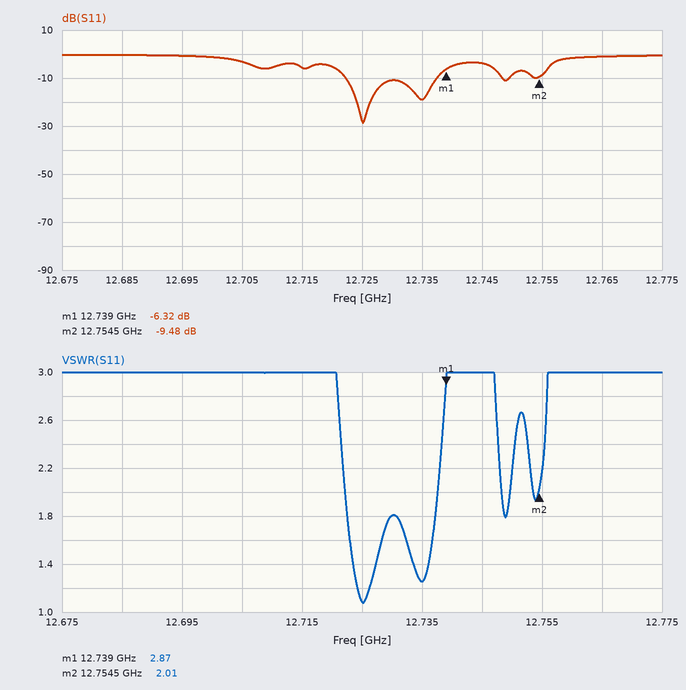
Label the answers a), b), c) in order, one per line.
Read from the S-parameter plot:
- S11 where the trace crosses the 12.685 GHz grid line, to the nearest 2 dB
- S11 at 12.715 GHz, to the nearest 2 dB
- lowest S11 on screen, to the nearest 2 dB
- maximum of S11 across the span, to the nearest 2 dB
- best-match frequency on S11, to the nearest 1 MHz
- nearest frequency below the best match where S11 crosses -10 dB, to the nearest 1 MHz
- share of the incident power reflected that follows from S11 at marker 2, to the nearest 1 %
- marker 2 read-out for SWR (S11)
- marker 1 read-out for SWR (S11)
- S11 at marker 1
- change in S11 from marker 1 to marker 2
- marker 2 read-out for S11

a) 0 dB
b) -6 dB
c) -28 dB
d) 0 dB
e) 12.725 GHz
f) 12.722 GHz
g) 11 %
h) 2.01
i) 2.87
j) -6.32 dB
k) -3.16 dB
l) -9.48 dB
